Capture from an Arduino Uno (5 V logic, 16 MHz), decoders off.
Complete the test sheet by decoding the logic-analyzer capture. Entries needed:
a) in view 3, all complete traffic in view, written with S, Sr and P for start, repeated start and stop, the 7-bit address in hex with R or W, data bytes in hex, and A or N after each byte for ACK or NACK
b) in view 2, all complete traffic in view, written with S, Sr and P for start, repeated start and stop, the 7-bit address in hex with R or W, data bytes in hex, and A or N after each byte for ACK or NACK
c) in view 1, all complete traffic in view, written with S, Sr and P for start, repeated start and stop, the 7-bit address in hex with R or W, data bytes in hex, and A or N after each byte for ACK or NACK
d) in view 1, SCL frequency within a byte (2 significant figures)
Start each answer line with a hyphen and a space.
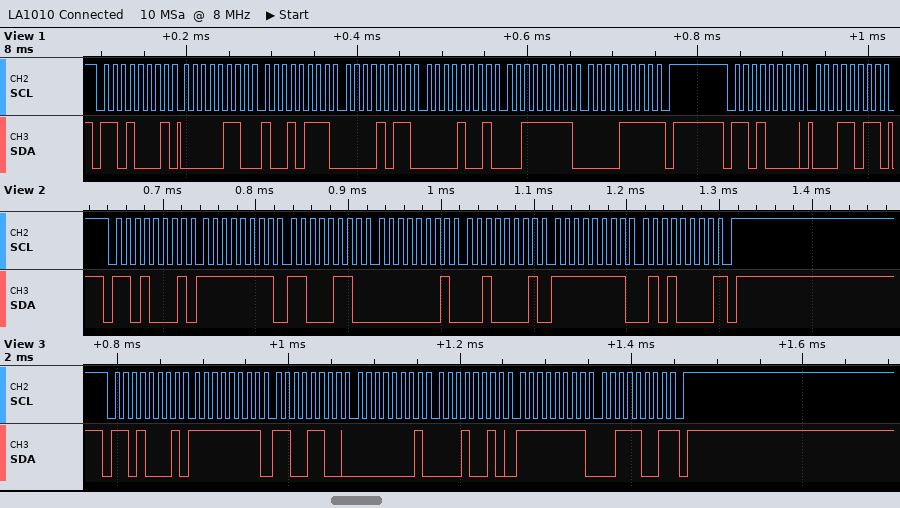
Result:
- S 68R A FF A CC A 01 A 12 A FF A 39 N P
- S 68R A FF A C6 A 01 A 21 A FF A 50 N P
- S 68R A 06 A 97 A 0B A 09 A 3F A 0F N P S 68W A 1B A
- 100 kHz
